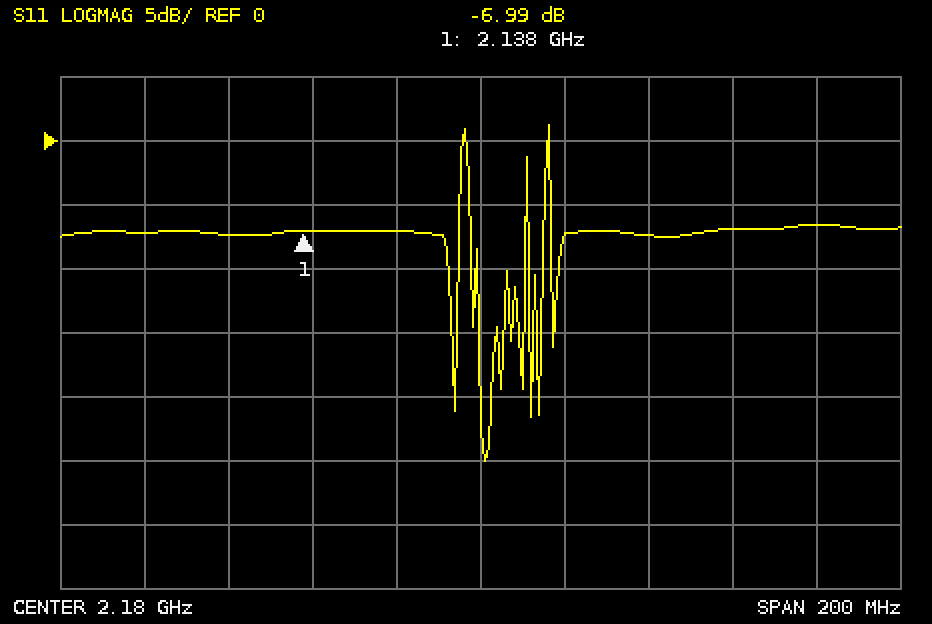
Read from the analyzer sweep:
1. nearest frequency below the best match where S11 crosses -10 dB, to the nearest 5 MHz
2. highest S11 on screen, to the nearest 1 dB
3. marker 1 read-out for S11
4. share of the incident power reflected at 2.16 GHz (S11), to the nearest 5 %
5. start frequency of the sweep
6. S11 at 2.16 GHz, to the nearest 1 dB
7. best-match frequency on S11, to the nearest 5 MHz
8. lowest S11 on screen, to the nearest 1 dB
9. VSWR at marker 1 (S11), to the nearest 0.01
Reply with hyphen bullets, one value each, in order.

- 2.180 GHz
- 1 dB
- -6.99 dB
- 20 %
- 2.08 GHz
- -7 dB
- 2.180 GHz
- -25 dB
- 2.62
